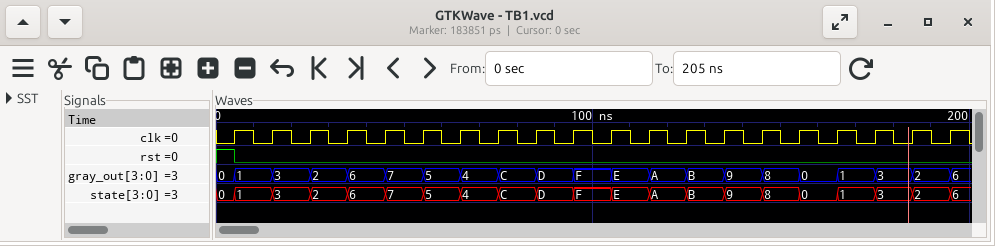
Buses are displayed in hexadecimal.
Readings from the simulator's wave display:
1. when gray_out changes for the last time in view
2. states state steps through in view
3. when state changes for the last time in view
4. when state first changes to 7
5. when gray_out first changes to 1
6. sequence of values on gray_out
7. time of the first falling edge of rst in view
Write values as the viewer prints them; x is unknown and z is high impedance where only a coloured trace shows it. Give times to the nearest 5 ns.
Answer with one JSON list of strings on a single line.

["195 ns", "0, 1, 3, 2, 6, 7, 5, 4, C, D, F, E, A, B, 9, 8, 0, 1, 3, 2, 6", "195 ns", "45 ns", "5 ns", "0, 1, 3, 2, 6, 7, 5, 4, C, D, F, E, A, B, 9, 8, 0, 1, 3, 2, 6", "5 ns"]
